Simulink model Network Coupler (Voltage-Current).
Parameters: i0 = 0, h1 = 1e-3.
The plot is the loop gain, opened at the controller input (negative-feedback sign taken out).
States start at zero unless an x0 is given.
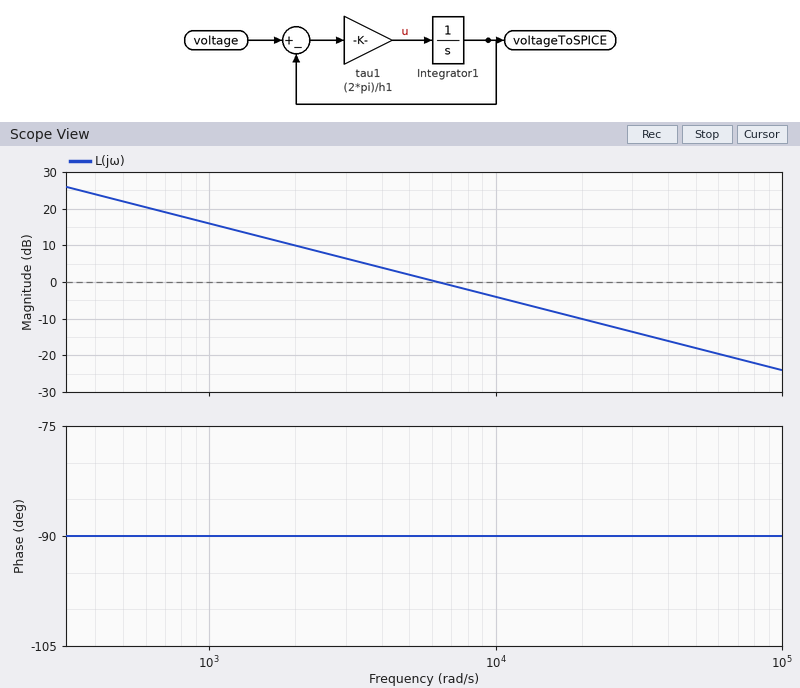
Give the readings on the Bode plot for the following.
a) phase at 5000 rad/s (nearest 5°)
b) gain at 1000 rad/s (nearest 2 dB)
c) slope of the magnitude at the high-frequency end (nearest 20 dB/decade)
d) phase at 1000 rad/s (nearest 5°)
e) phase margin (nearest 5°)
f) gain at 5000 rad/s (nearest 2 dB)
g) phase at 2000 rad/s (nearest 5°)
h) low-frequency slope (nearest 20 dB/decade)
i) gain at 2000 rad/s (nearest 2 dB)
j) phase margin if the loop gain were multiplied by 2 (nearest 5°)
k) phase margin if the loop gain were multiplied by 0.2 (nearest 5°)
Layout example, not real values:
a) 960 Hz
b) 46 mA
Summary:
a) -90°
b) 16 dB
c) -20 dB/decade
d) -90°
e) 90°
f) 2 dB
g) -90°
h) -20 dB/decade
i) 10 dB
j) 90°
k) 90°
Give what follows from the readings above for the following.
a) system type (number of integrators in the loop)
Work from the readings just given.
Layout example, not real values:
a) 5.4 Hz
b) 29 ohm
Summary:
a) 1
